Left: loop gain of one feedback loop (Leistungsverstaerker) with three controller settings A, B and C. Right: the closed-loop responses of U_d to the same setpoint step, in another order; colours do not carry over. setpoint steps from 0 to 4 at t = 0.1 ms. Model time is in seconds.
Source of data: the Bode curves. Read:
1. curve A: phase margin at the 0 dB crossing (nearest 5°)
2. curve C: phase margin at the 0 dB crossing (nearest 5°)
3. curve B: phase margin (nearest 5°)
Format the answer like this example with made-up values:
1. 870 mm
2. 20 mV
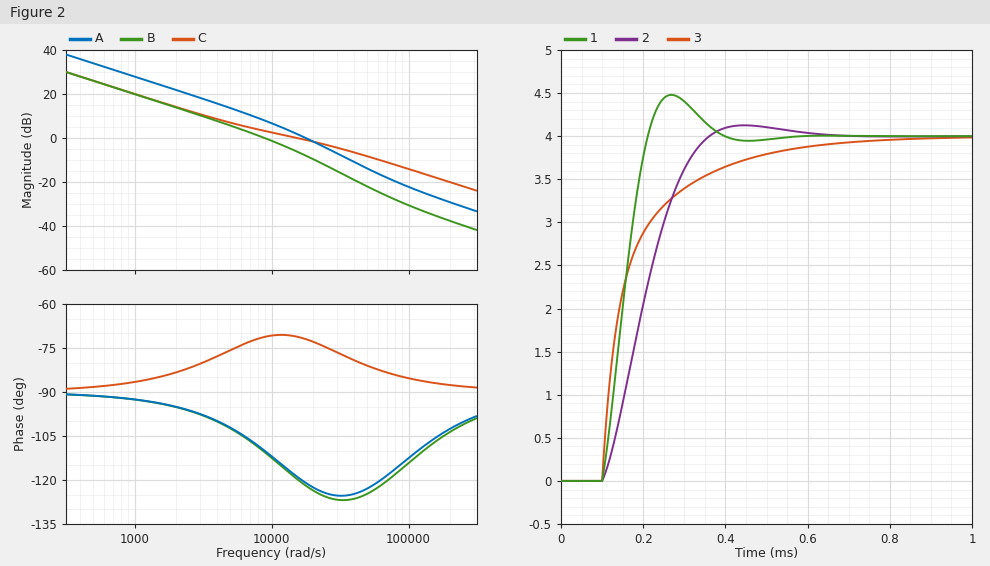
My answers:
1. 60°
2. 110°
3. 70°
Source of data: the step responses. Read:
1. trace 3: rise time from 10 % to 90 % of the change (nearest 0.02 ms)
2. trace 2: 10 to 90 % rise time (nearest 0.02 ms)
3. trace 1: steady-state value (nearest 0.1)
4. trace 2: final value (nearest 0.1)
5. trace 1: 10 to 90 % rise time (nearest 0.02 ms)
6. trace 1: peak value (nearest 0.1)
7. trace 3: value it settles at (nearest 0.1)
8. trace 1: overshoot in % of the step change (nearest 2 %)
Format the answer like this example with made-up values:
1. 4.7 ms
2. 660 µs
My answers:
1. 0.28 ms
2. 0.18 ms
3. 4.0
4. 4.0
5. 0.08 ms
6. 4.5
7. 4.0
8. 12 %
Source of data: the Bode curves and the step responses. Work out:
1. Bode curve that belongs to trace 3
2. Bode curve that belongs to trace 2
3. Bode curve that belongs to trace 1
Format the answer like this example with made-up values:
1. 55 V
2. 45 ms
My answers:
1. C
2. B
3. A
